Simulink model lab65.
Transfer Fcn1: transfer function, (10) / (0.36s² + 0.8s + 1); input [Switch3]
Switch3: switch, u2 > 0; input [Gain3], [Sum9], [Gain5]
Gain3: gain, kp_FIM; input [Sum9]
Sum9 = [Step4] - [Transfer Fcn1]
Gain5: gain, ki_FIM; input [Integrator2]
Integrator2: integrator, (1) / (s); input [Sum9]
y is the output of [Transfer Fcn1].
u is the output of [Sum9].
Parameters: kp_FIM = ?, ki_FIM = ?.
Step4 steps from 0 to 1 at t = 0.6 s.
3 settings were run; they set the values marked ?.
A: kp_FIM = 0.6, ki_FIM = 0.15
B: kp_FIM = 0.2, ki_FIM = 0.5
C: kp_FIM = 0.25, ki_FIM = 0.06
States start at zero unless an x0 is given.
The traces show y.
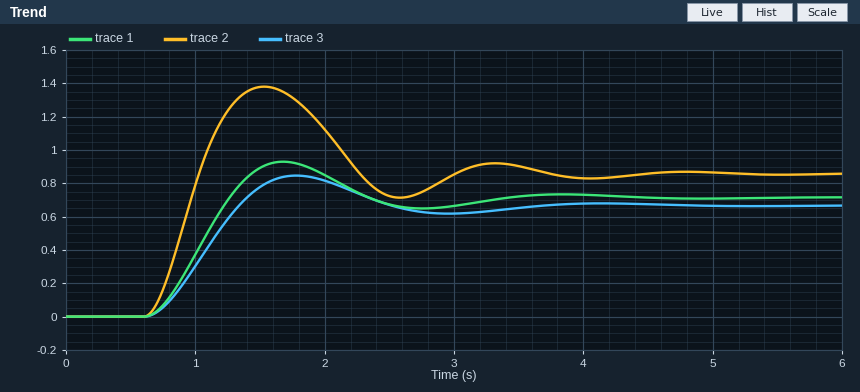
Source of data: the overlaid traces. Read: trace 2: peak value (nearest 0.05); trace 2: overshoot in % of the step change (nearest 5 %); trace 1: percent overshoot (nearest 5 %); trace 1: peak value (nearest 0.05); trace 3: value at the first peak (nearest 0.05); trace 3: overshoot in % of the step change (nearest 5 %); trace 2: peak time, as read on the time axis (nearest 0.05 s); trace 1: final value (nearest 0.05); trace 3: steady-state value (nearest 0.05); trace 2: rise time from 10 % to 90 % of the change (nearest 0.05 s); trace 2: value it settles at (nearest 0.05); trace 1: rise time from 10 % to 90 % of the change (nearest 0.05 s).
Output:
1.40
60 %
30 %
0.95
0.85
25 %
1.55 s
0.70
0.65
0.30 s
0.85
0.45 s
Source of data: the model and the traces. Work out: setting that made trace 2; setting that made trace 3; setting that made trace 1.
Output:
A
B
C
